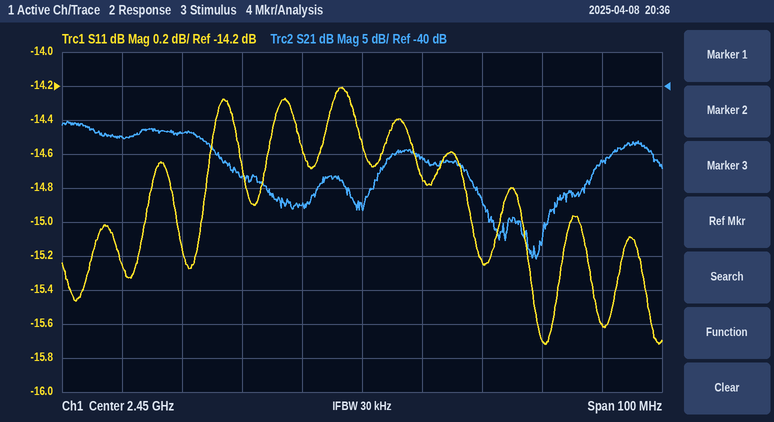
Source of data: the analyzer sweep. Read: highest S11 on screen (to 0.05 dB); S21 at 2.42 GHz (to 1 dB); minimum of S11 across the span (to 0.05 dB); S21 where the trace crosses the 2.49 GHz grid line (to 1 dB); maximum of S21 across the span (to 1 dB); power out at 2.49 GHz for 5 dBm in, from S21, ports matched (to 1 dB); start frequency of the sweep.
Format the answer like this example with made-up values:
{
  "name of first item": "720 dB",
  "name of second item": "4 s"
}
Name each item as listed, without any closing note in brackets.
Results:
{
  "highest S11 on screen": "-14.20 dB",
  "S21 at 2.42 GHz": "-47 dB",
  "minimum of S11 across the span": "-15.70 dB",
  "S21 where the trace crosses the 2.49 GHz grid line": "-51 dB",
  "maximum of S21 across the span": "-45 dB",
  "power out at 2.49 GHz for 5 dBm in, from S21, ports matched": "-46 dBm",
  "start frequency of the sweep": "2.4 GHz"
}
